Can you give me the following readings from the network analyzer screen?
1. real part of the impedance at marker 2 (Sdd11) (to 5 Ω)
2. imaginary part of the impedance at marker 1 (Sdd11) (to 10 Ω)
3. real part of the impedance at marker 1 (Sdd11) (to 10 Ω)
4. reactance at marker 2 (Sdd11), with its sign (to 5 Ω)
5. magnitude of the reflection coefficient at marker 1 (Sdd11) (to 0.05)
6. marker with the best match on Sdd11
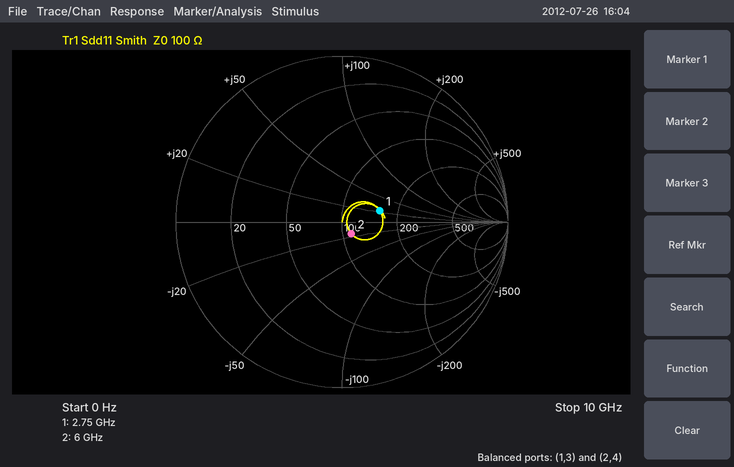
110 Ω
+20 Ω
160 Ω
-15 Ω
0.25
marker 2
